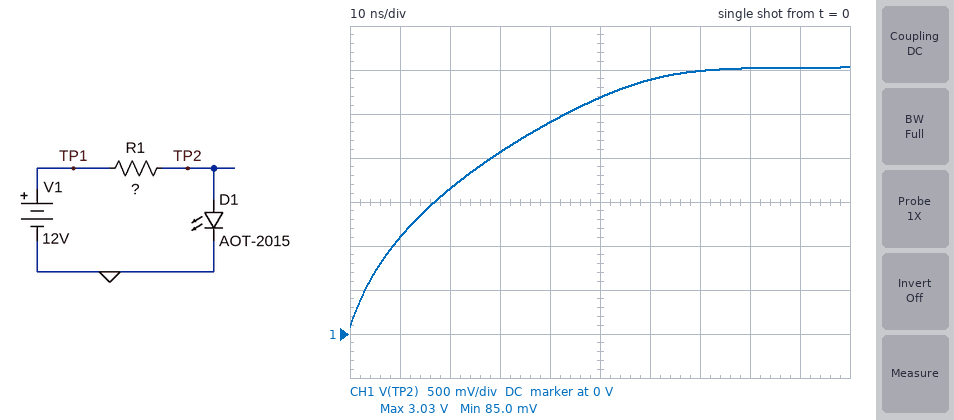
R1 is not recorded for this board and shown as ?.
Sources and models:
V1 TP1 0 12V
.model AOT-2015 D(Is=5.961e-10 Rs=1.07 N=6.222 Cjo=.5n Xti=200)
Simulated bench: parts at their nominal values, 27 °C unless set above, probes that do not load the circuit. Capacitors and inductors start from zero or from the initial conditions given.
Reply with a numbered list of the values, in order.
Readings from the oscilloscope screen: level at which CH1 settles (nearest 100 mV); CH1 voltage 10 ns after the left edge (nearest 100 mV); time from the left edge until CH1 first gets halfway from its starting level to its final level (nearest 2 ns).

1. 3.0 V
2. 1.1 V
3. 18 ns
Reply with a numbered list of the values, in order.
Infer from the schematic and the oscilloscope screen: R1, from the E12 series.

1. 150 Ω
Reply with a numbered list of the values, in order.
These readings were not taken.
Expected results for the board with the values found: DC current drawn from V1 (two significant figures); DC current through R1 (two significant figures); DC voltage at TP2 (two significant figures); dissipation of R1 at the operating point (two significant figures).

1. 60 mA
2. 60 mA
3. 3.0 V
4. 540 mW
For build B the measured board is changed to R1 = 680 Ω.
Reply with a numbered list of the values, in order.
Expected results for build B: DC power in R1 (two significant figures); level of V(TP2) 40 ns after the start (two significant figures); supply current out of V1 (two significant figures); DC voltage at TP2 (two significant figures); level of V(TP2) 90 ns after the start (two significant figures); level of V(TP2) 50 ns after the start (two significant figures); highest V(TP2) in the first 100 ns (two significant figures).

1. 130 mW
2. 960 mV
3. 14 mA
4. 2.7 V
5. 1.6 V
6. 1.1 V
7. 1.7 V
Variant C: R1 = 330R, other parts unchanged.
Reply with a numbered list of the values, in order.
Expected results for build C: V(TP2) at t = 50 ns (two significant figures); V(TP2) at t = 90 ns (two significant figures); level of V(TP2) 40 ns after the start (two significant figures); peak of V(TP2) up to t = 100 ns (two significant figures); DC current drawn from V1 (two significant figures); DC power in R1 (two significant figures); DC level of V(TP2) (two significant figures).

1. 1.7 V
2. 2.4 V
3. 1.5 V
4. 2.5 V
5. 28 mA
6. 250 mW
7. 2.9 V
